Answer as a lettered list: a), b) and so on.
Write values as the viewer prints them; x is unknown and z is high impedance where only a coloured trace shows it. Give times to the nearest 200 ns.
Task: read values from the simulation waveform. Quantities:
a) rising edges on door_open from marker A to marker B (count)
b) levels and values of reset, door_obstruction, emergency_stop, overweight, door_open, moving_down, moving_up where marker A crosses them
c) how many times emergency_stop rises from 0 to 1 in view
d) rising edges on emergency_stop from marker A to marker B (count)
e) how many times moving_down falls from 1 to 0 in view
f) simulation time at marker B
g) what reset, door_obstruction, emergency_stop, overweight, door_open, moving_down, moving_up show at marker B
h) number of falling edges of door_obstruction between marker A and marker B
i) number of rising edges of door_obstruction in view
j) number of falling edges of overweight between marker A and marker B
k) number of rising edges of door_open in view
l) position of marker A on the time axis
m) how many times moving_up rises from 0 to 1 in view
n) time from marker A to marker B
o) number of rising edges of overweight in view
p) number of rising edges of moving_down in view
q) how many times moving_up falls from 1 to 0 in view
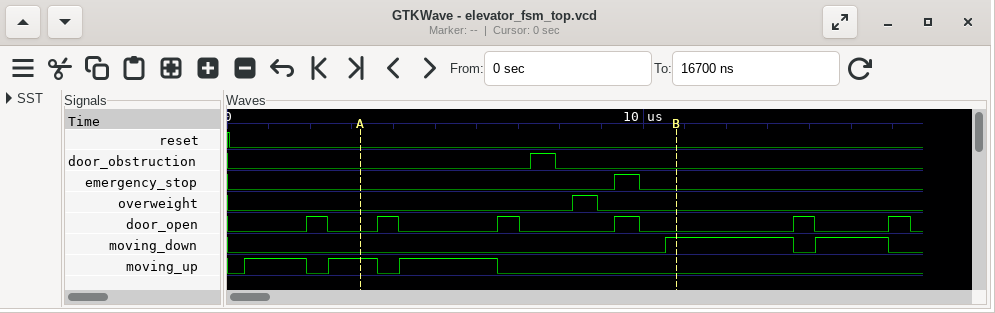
a) 3
b) reset=0, door_obstruction=0, emergency_stop=0, overweight=0, door_open=0, moving_down=0, moving_up=1
c) 1
d) 1
e) 2
f) 10800 ns
g) reset=0, door_obstruction=0, emergency_stop=0, overweight=0, door_open=0, moving_down=1, moving_up=0
h) 1
i) 1
j) 1
k) 6
l) 3200 ns
m) 3
n) 7600 ns
o) 1
p) 2
q) 3
